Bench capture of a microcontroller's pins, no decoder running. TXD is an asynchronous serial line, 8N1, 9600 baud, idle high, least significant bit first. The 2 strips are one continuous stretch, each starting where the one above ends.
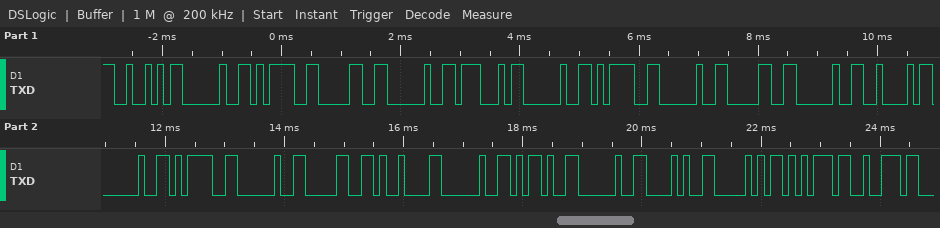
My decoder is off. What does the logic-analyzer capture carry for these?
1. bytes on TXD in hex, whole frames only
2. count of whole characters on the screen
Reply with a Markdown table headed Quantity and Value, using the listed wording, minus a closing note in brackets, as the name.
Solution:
| Quantity | Value |
|---|---|
| bytes on TXD in hex, whole frames only | 52 20 3D 30 20 47 20 3D 20 30 20 42 20 3D 20 30 09 20 2D 20 28 50 75 72 |
| count of whole characters on the screen | 24 |
